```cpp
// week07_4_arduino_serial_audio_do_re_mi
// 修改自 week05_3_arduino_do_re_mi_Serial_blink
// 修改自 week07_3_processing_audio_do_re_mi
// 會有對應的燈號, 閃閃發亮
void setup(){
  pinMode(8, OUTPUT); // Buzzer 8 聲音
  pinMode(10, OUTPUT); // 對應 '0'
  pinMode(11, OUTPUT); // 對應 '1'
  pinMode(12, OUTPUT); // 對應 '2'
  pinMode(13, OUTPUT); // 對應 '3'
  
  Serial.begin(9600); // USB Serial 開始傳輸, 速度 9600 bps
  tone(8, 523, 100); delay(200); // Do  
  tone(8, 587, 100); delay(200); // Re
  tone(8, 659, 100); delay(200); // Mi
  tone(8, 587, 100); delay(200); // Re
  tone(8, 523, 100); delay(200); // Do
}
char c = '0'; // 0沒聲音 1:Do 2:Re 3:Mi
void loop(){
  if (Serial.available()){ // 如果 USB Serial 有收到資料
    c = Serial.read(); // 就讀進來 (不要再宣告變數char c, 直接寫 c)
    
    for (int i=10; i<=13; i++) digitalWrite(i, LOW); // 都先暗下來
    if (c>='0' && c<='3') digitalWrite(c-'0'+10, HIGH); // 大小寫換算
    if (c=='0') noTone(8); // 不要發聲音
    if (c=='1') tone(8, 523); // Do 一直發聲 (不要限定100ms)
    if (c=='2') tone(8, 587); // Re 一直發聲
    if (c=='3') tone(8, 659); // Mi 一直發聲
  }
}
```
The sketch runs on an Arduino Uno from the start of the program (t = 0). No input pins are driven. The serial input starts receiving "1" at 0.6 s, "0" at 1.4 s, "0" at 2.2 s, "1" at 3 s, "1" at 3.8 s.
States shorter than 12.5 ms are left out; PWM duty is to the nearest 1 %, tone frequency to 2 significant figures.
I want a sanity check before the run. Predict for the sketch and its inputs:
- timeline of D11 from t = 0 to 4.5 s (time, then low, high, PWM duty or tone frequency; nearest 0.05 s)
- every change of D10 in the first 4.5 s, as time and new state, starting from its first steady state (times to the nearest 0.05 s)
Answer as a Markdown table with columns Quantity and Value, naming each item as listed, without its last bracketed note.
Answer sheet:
| Quantity | Value |
|---|---|
| timeline of D11 from t = 0 to 4.5 s | 0 s low; 1 s high; 1.4 s low; 3 s high |
| every change of D10 in the first 4.5 s, as time and new state, starting from its first steady state | 0 s low; 1.4 s high; 3 s low |
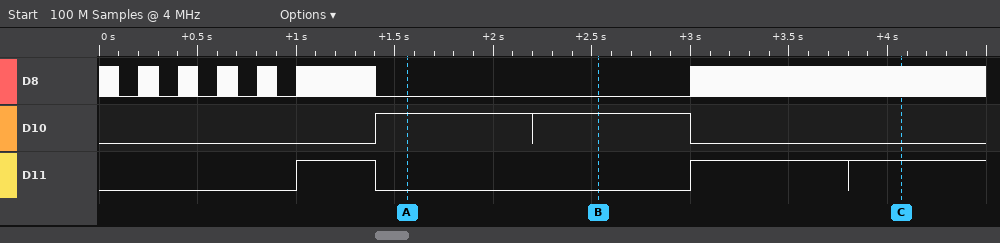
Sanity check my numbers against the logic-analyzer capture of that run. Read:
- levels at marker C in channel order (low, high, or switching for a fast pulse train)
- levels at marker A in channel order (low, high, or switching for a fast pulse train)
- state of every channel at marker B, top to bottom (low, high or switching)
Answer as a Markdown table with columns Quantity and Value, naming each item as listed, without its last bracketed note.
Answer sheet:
| Quantity | Value |
|---|---|
| levels at marker C in channel order | D8 switching, D10 low, D11 high |
| levels at marker A in channel order | D8 low, D10 high, D11 low |
| state of every channel at marker B, top to bottom | D8 low, D10 high, D11 low |
